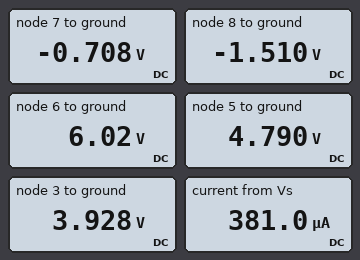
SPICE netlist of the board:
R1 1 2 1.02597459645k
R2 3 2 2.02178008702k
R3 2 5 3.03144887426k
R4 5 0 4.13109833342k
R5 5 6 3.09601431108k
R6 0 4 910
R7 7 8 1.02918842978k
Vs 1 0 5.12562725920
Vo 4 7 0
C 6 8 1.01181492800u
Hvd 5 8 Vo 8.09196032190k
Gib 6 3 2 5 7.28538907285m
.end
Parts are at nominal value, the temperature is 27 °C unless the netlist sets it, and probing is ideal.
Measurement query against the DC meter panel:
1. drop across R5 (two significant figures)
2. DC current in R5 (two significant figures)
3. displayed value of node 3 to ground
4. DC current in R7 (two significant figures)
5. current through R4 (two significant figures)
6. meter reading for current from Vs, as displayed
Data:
1.2 V
400 µA
3.928 V
780 µA
1.2 mA
381.0 µA
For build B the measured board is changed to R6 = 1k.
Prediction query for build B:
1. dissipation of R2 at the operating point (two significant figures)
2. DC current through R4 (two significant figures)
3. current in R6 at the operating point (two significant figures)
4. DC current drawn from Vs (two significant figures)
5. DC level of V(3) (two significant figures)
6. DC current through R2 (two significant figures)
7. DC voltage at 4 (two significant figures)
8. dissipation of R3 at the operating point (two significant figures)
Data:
300 µW
1.2 mA
790 µA
370 µA
4.0 V
390 µA
-790 mV
930 nW
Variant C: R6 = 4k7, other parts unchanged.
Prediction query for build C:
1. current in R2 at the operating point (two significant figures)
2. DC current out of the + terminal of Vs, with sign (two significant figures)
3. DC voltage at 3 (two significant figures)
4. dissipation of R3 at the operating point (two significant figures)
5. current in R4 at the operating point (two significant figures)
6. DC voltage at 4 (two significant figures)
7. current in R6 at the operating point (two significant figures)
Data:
1.2 mA
-1.1 mA
8.6 V
8.3 µW
1.5 mA
-12 V
2.6 mA
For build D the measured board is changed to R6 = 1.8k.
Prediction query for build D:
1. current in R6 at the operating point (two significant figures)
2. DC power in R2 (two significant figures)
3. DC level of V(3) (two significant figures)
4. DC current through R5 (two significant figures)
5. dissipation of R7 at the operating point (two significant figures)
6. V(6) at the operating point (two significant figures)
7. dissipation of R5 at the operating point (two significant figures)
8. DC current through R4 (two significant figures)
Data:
930 µA
140 µW
4.3 V
270 µA
890 µW
5.7 V
220 µW
1.2 mA
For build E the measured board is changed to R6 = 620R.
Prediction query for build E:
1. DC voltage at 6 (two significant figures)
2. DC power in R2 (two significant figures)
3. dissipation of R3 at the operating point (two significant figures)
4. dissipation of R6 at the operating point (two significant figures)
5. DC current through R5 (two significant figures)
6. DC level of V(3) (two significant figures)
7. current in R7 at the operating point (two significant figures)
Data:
6.1 V
380 µW
1.2 µW
340 µW
430 µA
3.8 V
740 µA
